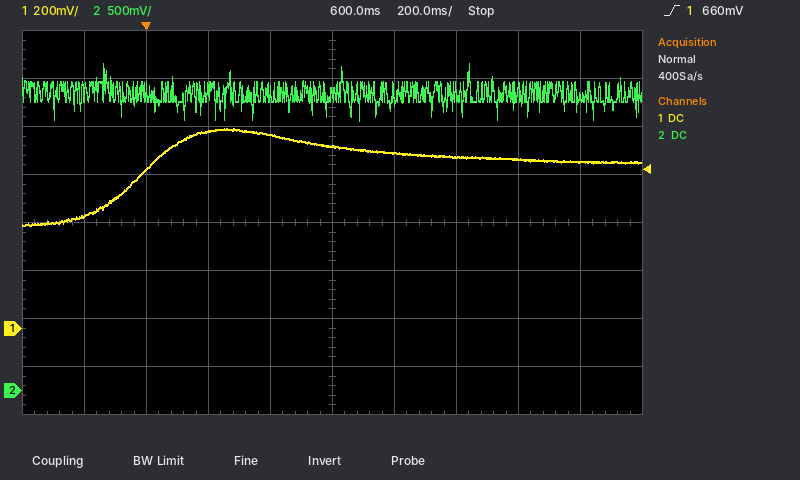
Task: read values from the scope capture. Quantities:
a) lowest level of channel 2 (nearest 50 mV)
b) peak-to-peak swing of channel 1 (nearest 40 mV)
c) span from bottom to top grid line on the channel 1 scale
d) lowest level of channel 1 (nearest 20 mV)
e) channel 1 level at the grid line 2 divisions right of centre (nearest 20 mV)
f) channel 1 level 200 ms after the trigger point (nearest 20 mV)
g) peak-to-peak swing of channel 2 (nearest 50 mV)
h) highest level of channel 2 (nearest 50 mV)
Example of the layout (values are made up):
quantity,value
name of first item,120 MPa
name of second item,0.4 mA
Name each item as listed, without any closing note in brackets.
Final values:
quantity,value
lowest level of channel 2,2.80 V
peak-to-peak swing of channel 1,400 mV
span from bottom to top grid line on the channel 1 scale,1.6 V
lowest level of channel 1,420 mV
channel 1 level at the grid line 2 divisions right of centre,720 mV
channel 1 level 200 ms after the trigger point,820 mV
peak-to-peak swing of channel 2,600 mV
highest level of channel 2,3.40 V
